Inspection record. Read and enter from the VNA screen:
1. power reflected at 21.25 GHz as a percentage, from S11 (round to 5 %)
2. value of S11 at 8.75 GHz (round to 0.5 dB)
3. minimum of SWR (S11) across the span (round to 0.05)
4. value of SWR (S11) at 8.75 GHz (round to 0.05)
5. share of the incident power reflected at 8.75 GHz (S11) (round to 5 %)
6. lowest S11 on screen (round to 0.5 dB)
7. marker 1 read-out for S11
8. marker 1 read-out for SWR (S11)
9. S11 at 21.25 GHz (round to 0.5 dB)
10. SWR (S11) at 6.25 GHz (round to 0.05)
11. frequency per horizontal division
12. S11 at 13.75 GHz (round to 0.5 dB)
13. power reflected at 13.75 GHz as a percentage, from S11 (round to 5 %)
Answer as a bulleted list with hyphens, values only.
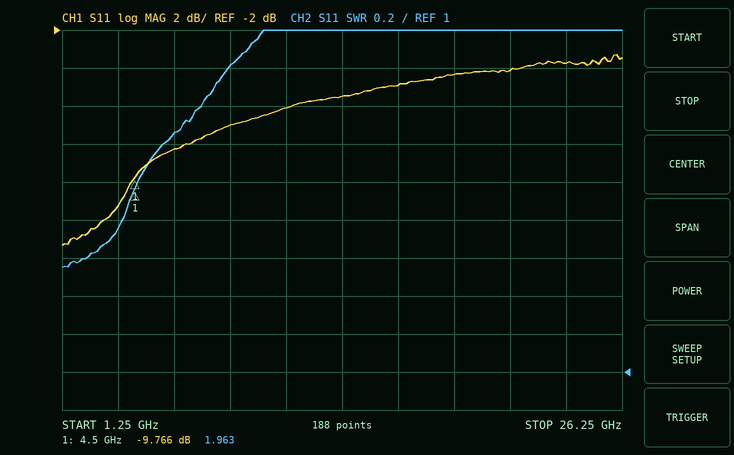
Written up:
- 40 %
- -7.0 dB
- 1.55
- 2.60
- 20 %
- -13.5 dB
- -9.766 dB
- 1.963
- -4.0 dB
- 2.25
- 2.5 GHz
- -5.5 dB
- 30 %
